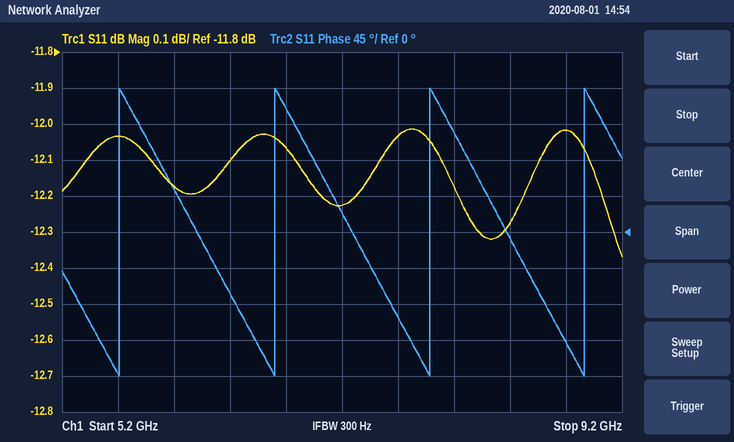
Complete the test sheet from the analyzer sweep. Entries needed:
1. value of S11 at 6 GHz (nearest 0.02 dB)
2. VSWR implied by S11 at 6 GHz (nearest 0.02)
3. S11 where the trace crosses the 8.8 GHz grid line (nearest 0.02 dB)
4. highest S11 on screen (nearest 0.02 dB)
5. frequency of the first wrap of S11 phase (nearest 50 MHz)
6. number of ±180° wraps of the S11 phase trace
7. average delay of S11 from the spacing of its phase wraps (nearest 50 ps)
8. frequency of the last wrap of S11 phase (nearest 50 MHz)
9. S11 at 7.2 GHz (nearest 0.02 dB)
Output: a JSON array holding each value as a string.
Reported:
["-12.18 dB", "1.66", "-12.02 dB", "-12.02 dB", "5.60 GHz", "4", "900 ps", "8.95 GHz", "-12.22 dB"]
